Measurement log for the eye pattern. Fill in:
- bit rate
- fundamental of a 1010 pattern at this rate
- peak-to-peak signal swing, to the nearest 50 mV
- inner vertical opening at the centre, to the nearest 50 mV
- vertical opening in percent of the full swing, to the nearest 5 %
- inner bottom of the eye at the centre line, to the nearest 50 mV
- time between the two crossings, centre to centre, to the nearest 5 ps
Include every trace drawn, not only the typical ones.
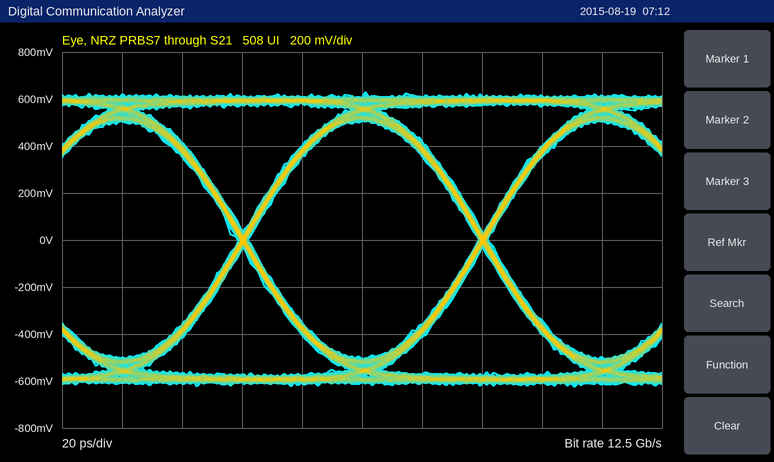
12.5 Gb/s
6.25 GHz
1.25 V
1.00 V
80 %
-500 mV
80 ps
